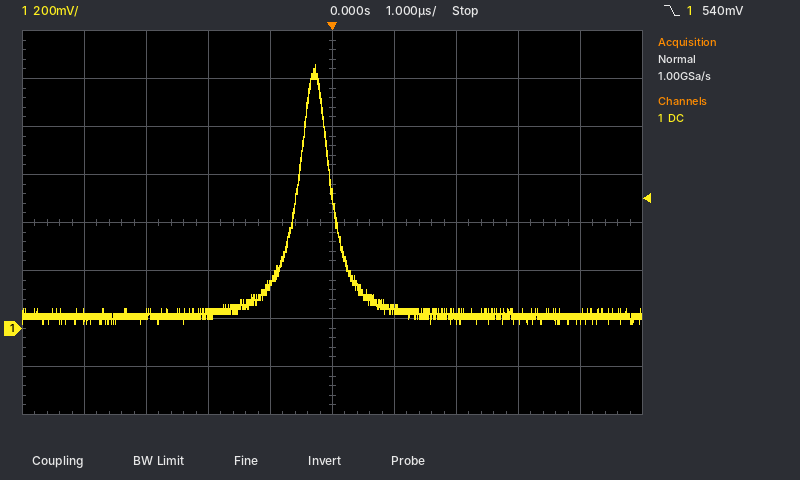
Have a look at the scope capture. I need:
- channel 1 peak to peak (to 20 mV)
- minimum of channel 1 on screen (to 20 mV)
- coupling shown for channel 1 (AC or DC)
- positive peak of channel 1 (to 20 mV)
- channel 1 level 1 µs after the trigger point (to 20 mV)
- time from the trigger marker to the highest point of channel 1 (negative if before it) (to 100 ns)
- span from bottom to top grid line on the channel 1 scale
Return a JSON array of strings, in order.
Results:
["1.08 V", "20 mV", "DC", "1.10 V", "80 mV", "-300 ns", "1.6 V"]
